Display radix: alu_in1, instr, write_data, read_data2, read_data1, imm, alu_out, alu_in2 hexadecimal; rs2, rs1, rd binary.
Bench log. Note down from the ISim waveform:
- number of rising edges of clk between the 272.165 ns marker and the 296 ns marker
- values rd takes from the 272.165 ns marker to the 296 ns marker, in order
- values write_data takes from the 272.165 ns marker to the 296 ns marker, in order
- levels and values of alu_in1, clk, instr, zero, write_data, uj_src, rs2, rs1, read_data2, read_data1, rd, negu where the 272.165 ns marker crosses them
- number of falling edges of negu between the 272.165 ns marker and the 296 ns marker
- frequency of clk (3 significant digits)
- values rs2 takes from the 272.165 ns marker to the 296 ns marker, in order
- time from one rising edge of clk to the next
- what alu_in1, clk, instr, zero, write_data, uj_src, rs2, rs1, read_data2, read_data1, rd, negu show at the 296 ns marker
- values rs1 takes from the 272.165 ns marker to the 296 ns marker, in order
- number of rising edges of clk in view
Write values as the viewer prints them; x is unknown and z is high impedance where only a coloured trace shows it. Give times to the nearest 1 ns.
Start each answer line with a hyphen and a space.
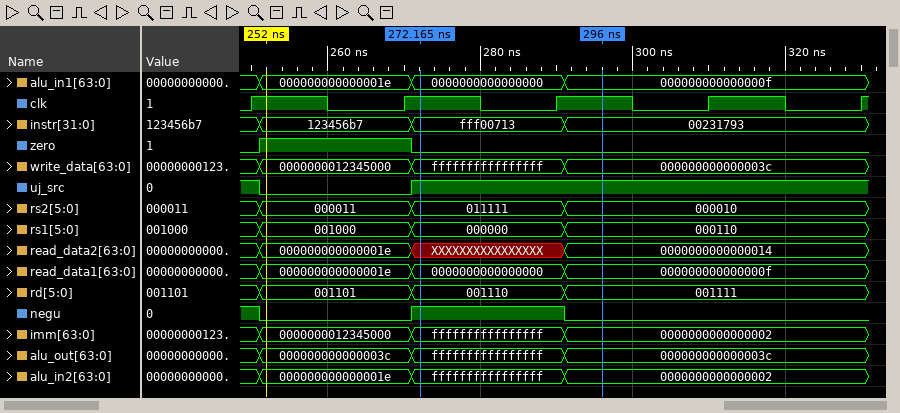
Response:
- 1
- 001110, 001111
- ffffffffffffffff, 000000000000003c
- alu_in1=0000000000000000, clk=1, instr=fff00713, zero=0, write_data=ffffffffffffffff, uj_src=1, rs2=011111, rs1=000000, read_data2=XXXXXXXXXXXXXXXX, read_data1=0000000000000000, rd=001110, negu=1
- 1
- 50.0 MHz
- 011111, 000010
- 20 ns
- alu_in1=000000000000000f, clk=1, instr=00231793, zero=0, write_data=000000000000003c, uj_src=1, rs2=000010, rs1=000110, read_data2=0000000000000014, read_data1=000000000000000f, rd=001111, negu=0
- 000000, 000110
- 5
